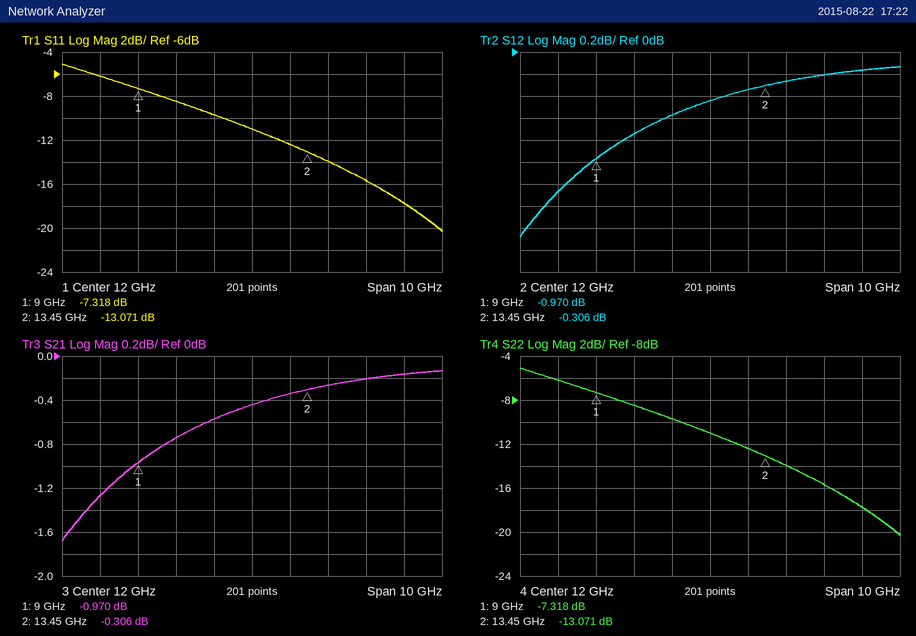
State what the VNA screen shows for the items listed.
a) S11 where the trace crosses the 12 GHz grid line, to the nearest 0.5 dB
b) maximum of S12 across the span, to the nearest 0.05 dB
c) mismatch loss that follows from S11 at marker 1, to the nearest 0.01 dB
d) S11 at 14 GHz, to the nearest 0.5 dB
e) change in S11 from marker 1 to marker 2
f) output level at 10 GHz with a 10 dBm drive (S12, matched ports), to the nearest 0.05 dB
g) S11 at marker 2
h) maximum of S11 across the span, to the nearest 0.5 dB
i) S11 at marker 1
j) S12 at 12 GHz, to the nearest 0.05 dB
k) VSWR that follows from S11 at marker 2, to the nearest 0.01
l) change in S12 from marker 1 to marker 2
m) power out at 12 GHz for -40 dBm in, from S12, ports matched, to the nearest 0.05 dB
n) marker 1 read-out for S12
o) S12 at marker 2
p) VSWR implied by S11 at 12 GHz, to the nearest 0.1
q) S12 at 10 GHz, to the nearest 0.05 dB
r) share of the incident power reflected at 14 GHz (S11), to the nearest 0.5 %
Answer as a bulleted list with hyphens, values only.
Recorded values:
- -11.0 dB
- -0.15 dB
- 0.89 dB
- -14.0 dB
- -5.753 dB
- 9.25 dBm
- -13.071 dB
- -5.0 dB
- -7.318 dB
- -0.45 dB
- 1.57
- 0.664 dB
- -40.45 dBm
- -0.970 dB
- -0.306 dB
- 1.8
- -0.75 dB
- 4.0 %
